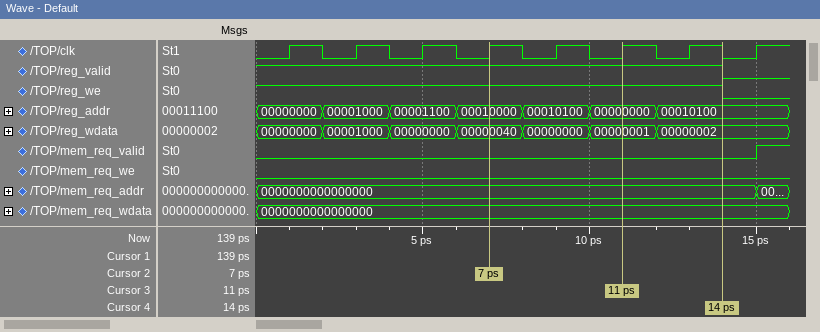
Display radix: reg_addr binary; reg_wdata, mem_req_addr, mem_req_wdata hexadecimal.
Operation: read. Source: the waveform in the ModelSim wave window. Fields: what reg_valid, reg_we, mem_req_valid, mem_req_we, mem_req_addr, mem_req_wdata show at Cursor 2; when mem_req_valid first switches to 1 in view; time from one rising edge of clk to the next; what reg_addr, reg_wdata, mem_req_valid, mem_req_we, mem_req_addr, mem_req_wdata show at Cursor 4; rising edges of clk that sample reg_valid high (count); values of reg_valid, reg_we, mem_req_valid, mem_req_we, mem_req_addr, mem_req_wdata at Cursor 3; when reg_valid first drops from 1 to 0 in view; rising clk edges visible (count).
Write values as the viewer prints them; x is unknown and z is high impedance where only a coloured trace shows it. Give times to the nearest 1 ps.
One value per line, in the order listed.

reg_valid=1, reg_we=1, mem_req_valid=0, mem_req_we=0, mem_req_addr=0000000000000000, mem_req_wdata=0000000000000000
15 ps
2 ps
reg_addr=00010100, reg_wdata=00000002, mem_req_valid=0, mem_req_we=0, mem_req_addr=0000000000000000, mem_req_wdata=0000000000000000
7
reg_valid=1, reg_we=1, mem_req_valid=0, mem_req_we=0, mem_req_addr=0000000000000000, mem_req_wdata=0000000000000000
14 ps
8
